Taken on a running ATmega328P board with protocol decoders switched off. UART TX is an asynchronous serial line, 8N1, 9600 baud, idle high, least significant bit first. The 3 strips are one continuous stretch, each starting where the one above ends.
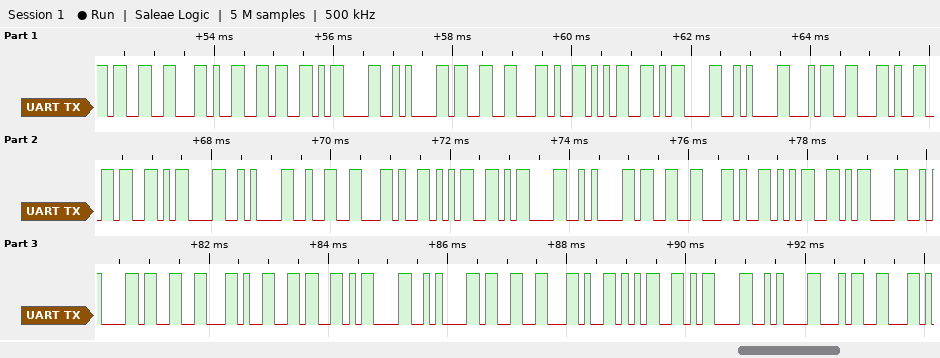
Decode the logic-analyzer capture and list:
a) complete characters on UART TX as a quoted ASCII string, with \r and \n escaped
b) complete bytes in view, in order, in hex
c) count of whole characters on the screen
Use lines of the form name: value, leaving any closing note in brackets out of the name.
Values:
complete characters on UART TX as a quoted ASCII string, with \r and \n escaped: "3,6\r\n3,5\r\n4,6\r\n2,5\r\n3,5\r\n3,6\r\n3,5\r\n4"
complete bytes in view, in order, in hex: 33 2C 36 0D 0A 33 2C 35 0D 0A 34 2C 36 0D 0A 32 2C 35 0D 0A 33 2C 35 0D 0A 33 2C 36 0D 0A 33 2C 35 0D 0A 34
count of whole characters on the screen: 36
